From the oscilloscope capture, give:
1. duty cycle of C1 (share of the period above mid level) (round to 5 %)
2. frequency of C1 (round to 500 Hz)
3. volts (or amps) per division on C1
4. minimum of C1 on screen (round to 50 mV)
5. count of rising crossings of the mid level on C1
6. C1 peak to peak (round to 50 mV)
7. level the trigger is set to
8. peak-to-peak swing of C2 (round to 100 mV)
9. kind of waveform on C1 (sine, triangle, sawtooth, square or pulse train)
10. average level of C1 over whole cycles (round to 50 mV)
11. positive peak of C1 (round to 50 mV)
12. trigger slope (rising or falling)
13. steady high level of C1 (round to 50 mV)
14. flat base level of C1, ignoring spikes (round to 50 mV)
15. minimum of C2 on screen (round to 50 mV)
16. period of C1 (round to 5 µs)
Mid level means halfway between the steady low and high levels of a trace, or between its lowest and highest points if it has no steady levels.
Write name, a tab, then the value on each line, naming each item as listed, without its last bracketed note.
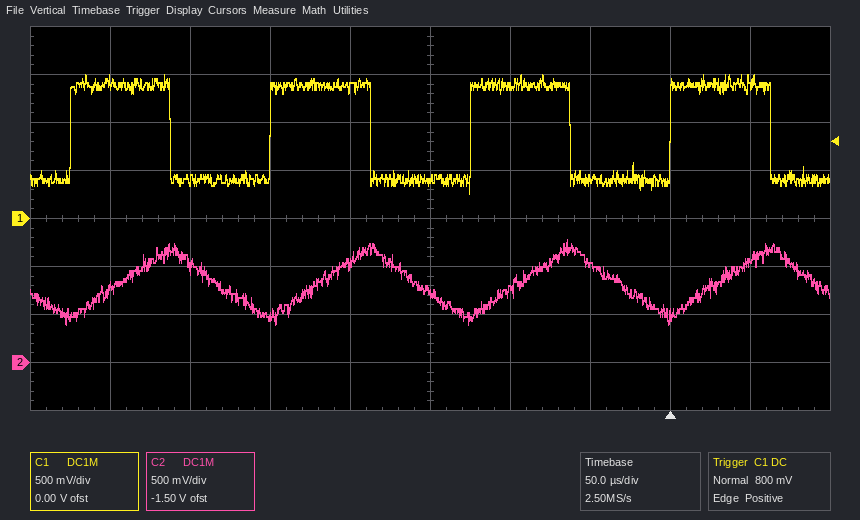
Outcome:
duty cycle of C1 (share of the period above mid level)	50 %
frequency of C1	8.0 kHz
volts (or amps) per division on C1	500 mV
minimum of C1 on screen	250 mV
count of rising crossings of the mid level on C1	4
C1 peak to peak	1.25 V
level the trigger is set to	800 mV
peak-to-peak swing of C2	900 mV
kind of waveform on C1	square
average level of C1 over whole cycles	900 mV
positive peak of C1	1.50 V
trigger slope	rising
steady high level of C1	1.40 V
flat base level of C1, ignoring spikes	400 mV
minimum of C2 on screen	400 mV
period of C1	125 µs
